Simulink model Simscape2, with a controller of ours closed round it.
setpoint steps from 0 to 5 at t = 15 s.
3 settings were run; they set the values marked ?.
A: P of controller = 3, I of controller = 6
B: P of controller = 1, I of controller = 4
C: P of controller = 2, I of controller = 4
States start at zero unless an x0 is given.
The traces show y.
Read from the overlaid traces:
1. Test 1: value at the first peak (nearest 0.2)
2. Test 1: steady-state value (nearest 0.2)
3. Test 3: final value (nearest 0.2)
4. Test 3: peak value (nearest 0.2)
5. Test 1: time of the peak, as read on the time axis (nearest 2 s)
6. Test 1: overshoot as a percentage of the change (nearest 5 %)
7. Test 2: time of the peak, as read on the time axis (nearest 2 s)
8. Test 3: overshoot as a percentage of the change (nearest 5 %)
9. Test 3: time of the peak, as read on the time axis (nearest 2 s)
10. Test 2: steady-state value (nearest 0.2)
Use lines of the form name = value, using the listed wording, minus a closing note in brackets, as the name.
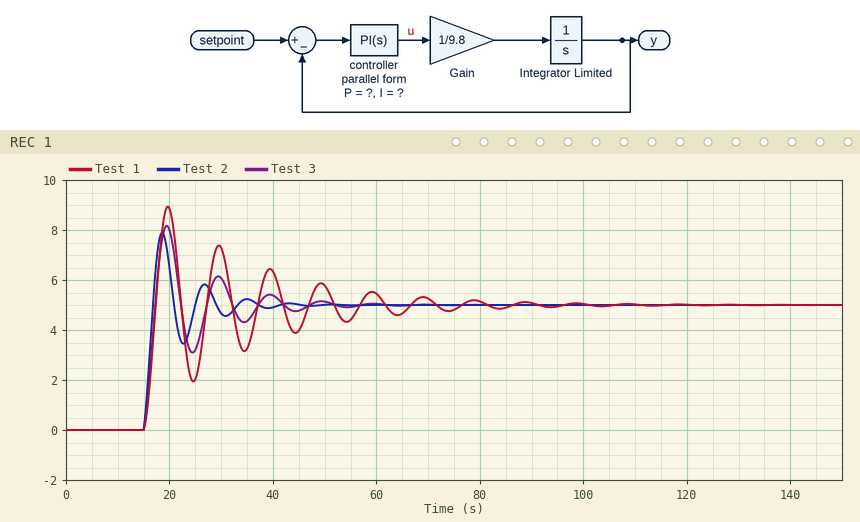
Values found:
Test 1: value at the first peak = 9.0
Test 1: steady-state value = 5.0
Test 3: final value = 5.0
Test 3: peak value = 8.2
Test 1: time of the peak, as read on the time axis = 20 s
Test 1: overshoot as a percentage of the change = 80 %
Test 2: time of the peak, as read on the time axis = 18 s
Test 3: overshoot as a percentage of the change = 65 %
Test 3: time of the peak, as read on the time axis = 20 s
Test 2: steady-state value = 5.0
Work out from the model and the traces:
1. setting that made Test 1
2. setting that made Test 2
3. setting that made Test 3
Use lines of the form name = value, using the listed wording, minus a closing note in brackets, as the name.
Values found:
setting that made Test 1 = B
setting that made Test 2 = A
setting that made Test 3 = C
